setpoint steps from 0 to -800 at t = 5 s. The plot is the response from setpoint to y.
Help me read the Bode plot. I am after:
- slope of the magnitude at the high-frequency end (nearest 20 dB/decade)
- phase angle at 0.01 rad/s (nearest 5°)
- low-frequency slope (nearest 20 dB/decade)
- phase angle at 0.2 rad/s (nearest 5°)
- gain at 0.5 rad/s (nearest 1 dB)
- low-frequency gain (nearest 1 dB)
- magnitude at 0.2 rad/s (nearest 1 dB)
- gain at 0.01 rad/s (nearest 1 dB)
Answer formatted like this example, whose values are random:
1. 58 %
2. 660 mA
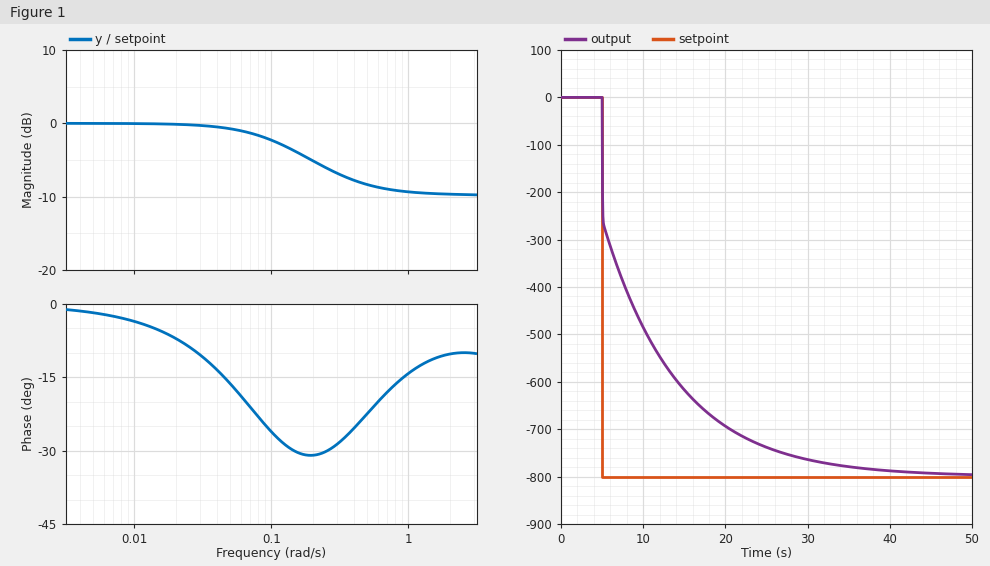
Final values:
1. 0 dB/decade
2. -5°
3. 0 dB/decade
4. -30°
5. -8 dB
6. 0 dB
7. -5 dB
8. 0 dB
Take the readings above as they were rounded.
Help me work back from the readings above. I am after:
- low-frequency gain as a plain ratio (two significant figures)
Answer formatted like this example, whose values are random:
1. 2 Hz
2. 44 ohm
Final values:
1. 1.0
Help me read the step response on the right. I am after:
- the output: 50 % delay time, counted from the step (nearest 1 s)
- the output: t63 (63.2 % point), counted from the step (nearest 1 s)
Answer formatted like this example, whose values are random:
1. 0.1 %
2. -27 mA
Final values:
1. 3 s
2. 6 s
